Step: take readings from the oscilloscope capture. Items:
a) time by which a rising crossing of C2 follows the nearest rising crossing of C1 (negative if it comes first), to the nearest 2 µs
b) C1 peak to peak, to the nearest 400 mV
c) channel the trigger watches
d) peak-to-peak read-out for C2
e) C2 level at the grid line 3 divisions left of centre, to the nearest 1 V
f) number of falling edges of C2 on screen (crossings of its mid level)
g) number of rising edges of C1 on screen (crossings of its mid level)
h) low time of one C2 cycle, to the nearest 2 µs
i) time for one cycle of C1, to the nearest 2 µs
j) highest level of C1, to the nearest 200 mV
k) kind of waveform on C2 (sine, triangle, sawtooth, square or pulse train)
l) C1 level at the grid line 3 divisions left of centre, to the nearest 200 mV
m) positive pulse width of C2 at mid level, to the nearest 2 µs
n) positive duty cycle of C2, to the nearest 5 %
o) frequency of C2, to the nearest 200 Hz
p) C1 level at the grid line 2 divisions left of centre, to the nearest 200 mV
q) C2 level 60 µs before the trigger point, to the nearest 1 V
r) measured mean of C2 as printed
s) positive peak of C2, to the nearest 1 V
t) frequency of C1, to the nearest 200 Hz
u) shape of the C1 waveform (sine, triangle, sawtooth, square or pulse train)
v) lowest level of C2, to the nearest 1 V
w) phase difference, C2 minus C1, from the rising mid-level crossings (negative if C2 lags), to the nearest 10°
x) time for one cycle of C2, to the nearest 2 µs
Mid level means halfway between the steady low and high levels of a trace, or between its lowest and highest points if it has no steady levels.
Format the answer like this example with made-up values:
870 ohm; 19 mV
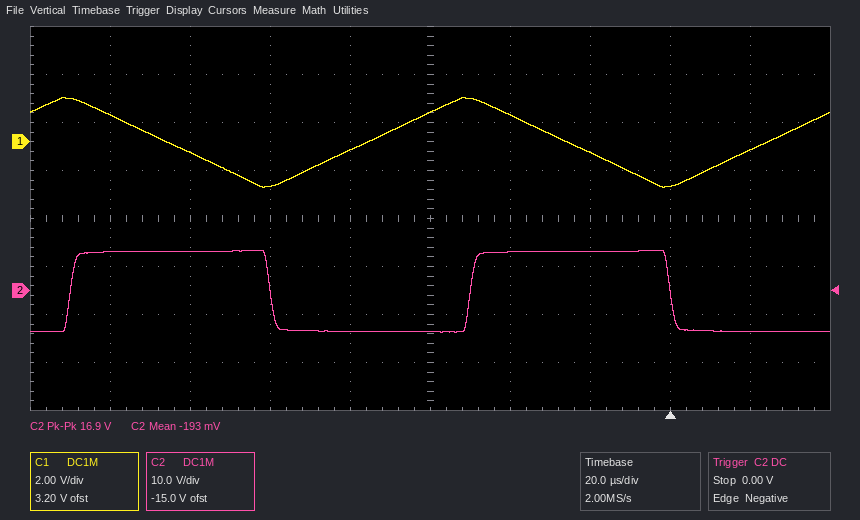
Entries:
+26 µs; 3.6 V; C2; 16.9 V; 8 V; 2; 2; 50 µs; 100 µs; 1.8 V; square; -400 mV; 50 µs; 50 %; 10.0 kHz; -1.8 V; -9 V; -193 mV; 8 V; 10.0 kHz; triangle; -9 V; -90°; 100 µs
